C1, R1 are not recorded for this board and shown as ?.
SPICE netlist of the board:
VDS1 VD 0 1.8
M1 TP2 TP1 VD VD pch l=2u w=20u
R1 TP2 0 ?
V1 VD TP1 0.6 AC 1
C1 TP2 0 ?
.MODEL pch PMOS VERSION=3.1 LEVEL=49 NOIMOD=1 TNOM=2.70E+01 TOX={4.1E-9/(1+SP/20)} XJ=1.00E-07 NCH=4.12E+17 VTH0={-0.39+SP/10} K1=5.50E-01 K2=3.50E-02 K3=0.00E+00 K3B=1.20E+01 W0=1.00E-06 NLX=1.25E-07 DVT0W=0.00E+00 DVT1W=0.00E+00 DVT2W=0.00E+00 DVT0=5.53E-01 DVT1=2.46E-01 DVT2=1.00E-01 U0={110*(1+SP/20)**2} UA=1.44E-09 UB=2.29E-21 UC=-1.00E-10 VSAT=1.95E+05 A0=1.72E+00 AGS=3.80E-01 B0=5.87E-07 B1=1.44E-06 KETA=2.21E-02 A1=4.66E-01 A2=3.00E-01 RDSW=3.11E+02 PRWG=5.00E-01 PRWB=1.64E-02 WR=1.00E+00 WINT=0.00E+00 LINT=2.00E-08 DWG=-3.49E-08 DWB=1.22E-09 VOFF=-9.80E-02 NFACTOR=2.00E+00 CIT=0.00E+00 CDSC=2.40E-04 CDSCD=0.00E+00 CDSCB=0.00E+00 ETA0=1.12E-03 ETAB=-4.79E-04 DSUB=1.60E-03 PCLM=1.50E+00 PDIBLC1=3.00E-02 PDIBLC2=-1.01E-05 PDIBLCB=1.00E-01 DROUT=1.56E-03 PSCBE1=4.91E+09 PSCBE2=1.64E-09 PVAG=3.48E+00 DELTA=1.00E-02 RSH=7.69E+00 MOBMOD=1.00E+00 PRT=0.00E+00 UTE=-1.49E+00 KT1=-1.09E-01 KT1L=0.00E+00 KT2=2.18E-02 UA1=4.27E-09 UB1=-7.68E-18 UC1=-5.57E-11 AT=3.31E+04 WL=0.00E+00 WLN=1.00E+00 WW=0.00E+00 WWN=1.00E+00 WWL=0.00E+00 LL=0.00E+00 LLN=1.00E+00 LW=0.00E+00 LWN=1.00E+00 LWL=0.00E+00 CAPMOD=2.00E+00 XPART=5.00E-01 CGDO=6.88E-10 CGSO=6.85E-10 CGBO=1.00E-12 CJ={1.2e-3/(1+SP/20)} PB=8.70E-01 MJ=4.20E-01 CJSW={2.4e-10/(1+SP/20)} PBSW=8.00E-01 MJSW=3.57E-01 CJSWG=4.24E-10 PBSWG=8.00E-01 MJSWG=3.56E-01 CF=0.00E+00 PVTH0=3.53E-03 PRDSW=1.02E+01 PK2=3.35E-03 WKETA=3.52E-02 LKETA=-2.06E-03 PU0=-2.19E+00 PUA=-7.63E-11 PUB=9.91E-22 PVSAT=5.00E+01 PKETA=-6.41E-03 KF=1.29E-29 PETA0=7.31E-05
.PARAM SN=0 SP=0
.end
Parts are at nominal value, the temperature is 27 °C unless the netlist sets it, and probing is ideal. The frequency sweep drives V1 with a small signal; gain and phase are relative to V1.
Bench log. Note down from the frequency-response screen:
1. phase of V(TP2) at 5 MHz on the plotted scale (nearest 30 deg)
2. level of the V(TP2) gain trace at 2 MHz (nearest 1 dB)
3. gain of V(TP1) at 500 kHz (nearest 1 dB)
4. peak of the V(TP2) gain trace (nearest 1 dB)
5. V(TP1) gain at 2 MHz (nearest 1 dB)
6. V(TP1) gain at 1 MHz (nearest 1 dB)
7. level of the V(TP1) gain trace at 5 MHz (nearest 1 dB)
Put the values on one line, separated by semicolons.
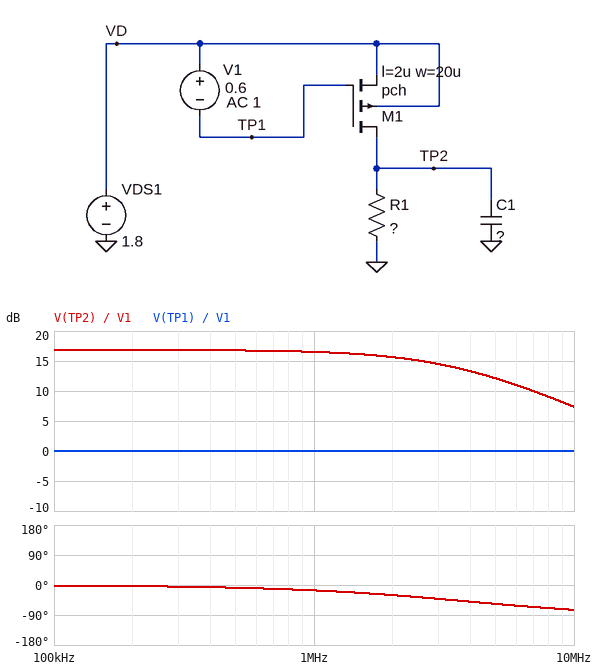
-60 deg; 16 dB; 0 dB; 17 dB; 0 dB; 0 dB; 0 dB
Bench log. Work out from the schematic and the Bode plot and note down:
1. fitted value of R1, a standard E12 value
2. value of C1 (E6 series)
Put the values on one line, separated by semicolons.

68 kΩ; 680 fF
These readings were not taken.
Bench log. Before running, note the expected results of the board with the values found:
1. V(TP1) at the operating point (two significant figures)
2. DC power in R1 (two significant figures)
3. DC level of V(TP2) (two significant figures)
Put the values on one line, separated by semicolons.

1.2 V; 8.9 µW; 780 mV
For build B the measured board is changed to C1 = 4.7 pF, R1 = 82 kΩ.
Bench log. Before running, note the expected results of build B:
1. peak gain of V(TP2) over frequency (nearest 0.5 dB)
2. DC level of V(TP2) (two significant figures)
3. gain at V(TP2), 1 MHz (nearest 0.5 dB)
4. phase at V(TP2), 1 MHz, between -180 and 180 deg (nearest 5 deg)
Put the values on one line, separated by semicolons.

18.5 dB; 930 mV; 10.5 dB; -65 deg
